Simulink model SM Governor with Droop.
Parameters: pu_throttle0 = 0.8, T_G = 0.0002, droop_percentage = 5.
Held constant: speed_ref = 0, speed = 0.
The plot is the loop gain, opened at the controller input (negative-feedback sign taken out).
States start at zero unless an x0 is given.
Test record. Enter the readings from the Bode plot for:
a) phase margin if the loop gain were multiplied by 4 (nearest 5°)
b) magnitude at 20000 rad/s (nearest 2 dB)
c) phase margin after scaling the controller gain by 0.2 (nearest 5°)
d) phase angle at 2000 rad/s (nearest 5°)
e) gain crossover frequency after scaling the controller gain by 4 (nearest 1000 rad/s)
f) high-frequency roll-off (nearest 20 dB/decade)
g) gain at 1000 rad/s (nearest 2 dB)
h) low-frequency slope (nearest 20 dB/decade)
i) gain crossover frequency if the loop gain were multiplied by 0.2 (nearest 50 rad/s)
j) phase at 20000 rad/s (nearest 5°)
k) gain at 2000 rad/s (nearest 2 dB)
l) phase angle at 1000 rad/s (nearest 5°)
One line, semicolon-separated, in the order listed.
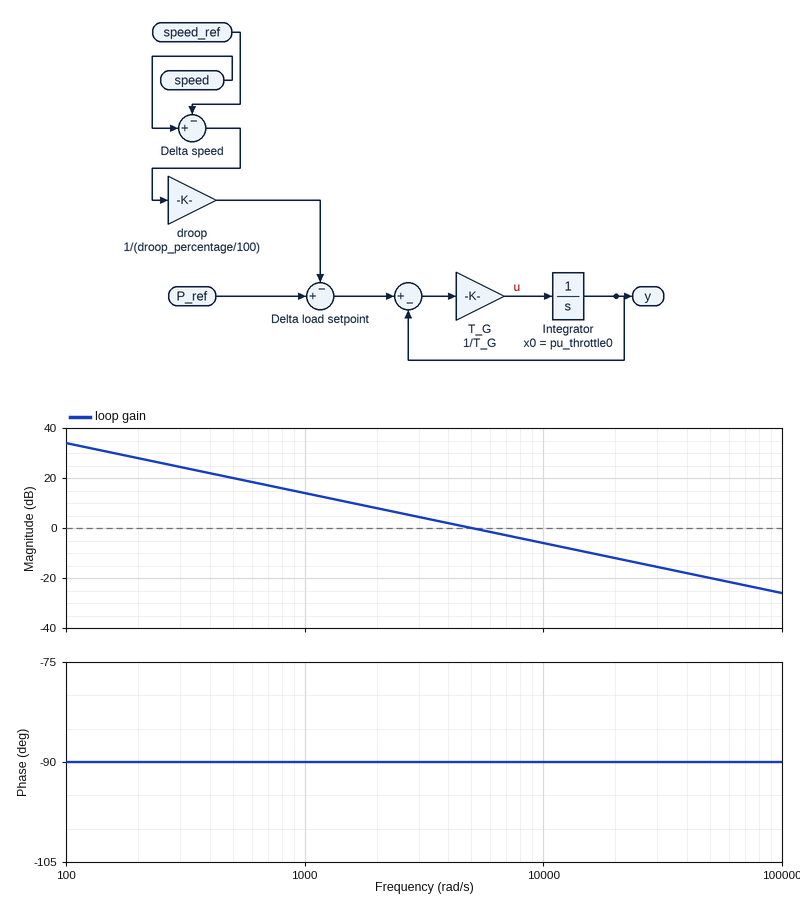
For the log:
90°; -12 dB; 90°; -90°; 20000 rad/s; -20 dB/decade; 14 dB; -20 dB/decade; 1000 rad/s; -90°; 8 dB; -90°
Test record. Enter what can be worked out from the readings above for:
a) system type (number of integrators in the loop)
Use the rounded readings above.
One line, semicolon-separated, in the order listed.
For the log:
1
